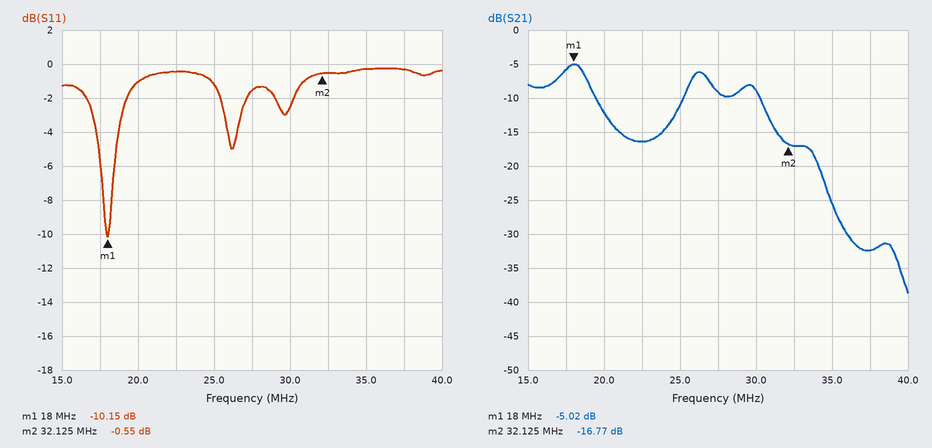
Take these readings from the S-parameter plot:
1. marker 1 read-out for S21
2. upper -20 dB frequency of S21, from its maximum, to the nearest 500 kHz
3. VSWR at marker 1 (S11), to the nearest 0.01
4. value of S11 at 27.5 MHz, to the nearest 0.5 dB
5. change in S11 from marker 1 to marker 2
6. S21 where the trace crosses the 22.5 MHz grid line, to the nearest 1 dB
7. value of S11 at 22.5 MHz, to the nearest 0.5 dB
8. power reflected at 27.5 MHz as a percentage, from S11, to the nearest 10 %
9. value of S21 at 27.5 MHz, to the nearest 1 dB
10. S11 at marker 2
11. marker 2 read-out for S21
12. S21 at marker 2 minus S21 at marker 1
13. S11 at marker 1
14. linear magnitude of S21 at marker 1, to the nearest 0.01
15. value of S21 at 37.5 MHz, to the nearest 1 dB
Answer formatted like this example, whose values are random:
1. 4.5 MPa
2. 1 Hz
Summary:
1. -5.02 dB
2. 35.0 MHz
3. 1.90
4. -1.5 dB
5. 9.60 dB
6. -16 dB
7. -0.5 dB
8. 70 %
9. -9 dB
10. -0.55 dB
11. -16.77 dB
12. -11.75 dB
13. -10.15 dB
14. 0.56
15. -32 dB
